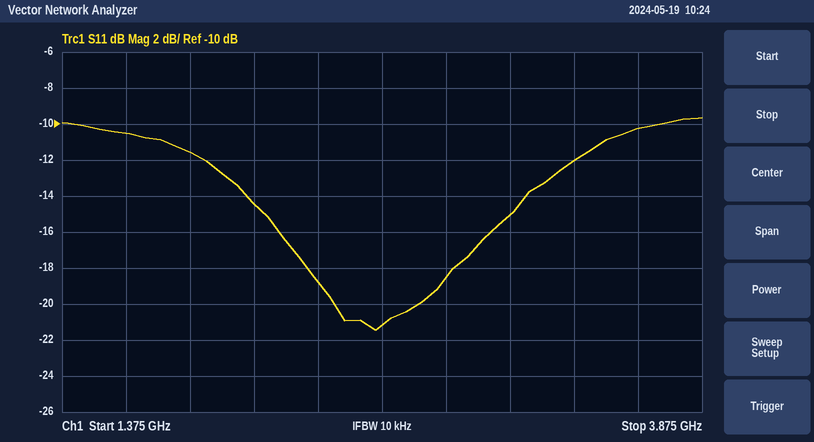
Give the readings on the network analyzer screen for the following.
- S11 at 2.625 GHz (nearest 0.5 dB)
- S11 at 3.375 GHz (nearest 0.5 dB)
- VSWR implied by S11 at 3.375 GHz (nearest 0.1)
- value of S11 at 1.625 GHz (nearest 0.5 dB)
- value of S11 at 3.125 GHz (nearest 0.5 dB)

-21.0 dB
-12.0 dB
1.7
-10.5 dB
-15.0 dB
